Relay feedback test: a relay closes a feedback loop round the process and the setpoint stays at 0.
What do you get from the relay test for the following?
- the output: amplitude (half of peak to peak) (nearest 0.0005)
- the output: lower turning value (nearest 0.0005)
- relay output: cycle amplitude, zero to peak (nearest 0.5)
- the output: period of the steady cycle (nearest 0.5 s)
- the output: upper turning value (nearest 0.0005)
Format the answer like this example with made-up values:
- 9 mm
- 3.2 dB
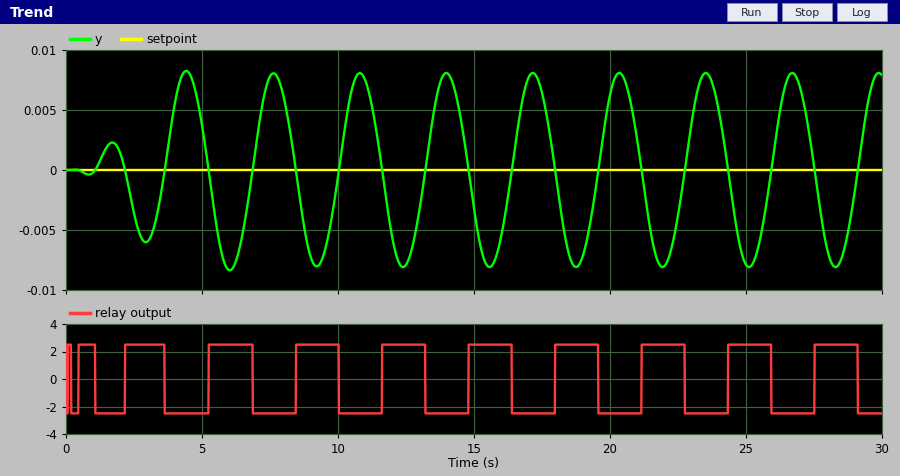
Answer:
- 0.0080
- -0.0080
- 2.5
- 3.0 s
- 0.0080
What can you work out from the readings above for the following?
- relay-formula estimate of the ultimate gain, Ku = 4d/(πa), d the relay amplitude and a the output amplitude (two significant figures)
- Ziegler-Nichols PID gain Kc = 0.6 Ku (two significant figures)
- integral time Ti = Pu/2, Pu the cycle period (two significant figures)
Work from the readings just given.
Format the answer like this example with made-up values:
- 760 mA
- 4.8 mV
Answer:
- 400
- 240
- 1.5 s
